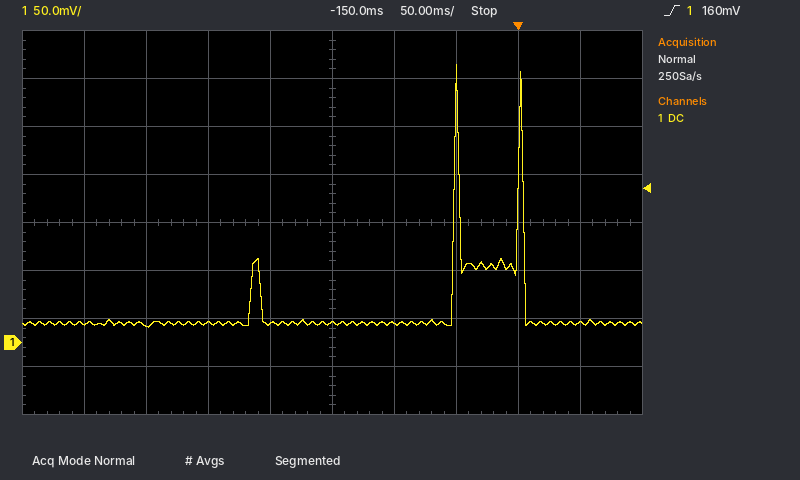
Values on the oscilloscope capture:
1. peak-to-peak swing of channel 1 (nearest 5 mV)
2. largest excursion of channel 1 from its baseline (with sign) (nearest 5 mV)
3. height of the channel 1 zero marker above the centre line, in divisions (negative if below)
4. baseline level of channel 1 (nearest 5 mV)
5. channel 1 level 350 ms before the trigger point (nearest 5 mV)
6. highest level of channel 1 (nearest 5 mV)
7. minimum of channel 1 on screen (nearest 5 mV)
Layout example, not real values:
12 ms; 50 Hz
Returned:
275 mV; +270 mV; -2.5 div; 20 mV; 20 mV; 290 mV; 15 mV
